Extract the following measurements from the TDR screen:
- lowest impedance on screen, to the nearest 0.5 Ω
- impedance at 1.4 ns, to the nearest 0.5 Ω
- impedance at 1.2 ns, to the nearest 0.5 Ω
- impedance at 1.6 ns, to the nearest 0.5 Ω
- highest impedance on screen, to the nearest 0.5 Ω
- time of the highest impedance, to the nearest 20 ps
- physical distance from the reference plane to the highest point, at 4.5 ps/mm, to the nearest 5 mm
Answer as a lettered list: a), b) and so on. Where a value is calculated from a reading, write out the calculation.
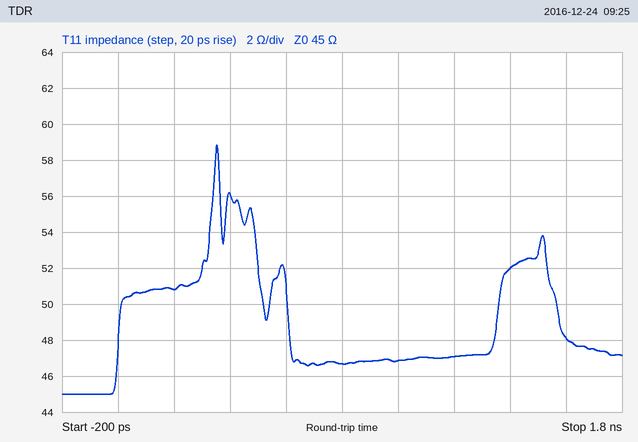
a) 45.0 Ω
b) 52.0 Ω
c) 47.0 Ω
d) 48.0 Ω
e) 59.0 Ω
f) 360 ps
g) 360 ps / 2 / 4.5 ps/mm ≈ 40 mm
